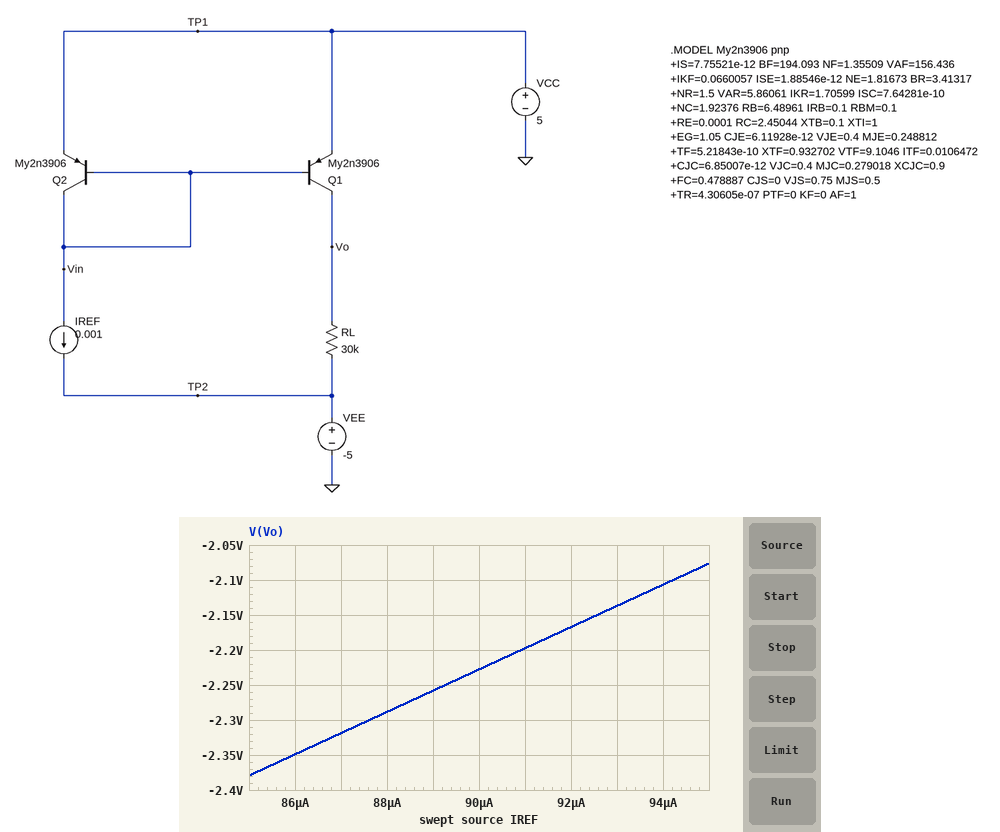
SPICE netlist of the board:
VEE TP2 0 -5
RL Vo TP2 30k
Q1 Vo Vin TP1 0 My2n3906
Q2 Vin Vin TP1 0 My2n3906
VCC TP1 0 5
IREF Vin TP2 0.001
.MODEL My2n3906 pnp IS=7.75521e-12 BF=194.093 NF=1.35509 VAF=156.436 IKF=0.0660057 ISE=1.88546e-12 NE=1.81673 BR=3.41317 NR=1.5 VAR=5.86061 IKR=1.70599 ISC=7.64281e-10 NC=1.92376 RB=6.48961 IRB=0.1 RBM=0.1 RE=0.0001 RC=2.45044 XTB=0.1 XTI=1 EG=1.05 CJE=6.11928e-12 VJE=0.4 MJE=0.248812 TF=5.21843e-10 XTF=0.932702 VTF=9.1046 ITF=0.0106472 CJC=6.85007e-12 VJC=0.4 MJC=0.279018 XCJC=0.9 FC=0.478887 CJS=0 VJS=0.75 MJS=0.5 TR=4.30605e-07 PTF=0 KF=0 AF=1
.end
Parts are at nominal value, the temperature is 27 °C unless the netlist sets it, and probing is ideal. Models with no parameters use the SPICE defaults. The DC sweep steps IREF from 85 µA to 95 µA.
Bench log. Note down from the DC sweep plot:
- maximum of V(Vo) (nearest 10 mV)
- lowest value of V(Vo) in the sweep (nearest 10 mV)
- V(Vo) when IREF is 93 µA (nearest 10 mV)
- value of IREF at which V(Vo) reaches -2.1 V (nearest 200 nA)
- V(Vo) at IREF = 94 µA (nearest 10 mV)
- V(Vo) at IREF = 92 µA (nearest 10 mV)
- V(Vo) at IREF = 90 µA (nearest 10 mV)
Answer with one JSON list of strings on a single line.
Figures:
["-2.08 V", "-2.38 V", "-2.14 V", "94.2 µA", "-2.11 V", "-2.17 V", "-2.23 V"]
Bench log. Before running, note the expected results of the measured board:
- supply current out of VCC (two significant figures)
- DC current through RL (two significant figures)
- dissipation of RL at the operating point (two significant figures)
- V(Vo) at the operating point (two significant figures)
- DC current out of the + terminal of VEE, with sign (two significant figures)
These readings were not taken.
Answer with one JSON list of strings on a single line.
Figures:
["1.3 mA", "330 µA", "3.3 mW", "5.0 V", "-1.3 mA"]
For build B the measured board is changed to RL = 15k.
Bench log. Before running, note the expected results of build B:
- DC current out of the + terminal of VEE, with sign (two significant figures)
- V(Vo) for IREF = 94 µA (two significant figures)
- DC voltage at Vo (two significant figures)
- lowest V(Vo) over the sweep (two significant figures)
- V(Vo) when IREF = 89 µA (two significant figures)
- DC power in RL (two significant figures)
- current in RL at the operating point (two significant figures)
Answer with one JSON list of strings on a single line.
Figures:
["-1.7 mA", "-3.5 V", "4.9 V", "-3.7 V", "-3.6 V", "6.6 mW", "660 µA"]
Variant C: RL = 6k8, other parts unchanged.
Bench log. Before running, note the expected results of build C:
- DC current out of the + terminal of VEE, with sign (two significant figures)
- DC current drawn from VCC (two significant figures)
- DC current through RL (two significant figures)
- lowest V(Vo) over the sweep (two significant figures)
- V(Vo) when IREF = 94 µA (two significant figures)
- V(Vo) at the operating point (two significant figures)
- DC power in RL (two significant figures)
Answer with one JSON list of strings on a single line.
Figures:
["-2.0 mA", "2.0 mA", "1.0 mA", "-4.4 V", "-4.3 V", "1.8 V", "6.8 mW"]
